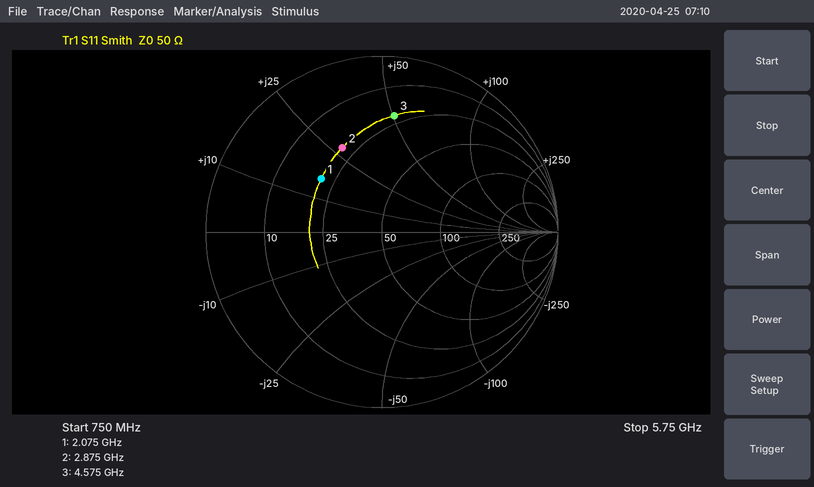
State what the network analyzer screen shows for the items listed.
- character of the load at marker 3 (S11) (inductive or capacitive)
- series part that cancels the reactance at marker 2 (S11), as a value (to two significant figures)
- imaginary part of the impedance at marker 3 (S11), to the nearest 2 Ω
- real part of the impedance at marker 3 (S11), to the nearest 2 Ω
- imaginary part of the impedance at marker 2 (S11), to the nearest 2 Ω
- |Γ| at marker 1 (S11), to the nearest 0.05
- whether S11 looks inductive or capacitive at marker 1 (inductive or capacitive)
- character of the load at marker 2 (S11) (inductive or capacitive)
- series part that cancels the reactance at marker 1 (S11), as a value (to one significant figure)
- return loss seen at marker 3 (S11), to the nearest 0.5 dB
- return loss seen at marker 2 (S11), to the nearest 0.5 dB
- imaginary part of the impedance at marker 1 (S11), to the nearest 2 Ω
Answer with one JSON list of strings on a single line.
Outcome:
["inductive", "2.0 pF", "+50 Ω", "22 Ω", "+28 Ω", "0.45", "inductive", "inductive", "5 pF", "3.5 dB", "5.5 dB", "+16 Ω"]
